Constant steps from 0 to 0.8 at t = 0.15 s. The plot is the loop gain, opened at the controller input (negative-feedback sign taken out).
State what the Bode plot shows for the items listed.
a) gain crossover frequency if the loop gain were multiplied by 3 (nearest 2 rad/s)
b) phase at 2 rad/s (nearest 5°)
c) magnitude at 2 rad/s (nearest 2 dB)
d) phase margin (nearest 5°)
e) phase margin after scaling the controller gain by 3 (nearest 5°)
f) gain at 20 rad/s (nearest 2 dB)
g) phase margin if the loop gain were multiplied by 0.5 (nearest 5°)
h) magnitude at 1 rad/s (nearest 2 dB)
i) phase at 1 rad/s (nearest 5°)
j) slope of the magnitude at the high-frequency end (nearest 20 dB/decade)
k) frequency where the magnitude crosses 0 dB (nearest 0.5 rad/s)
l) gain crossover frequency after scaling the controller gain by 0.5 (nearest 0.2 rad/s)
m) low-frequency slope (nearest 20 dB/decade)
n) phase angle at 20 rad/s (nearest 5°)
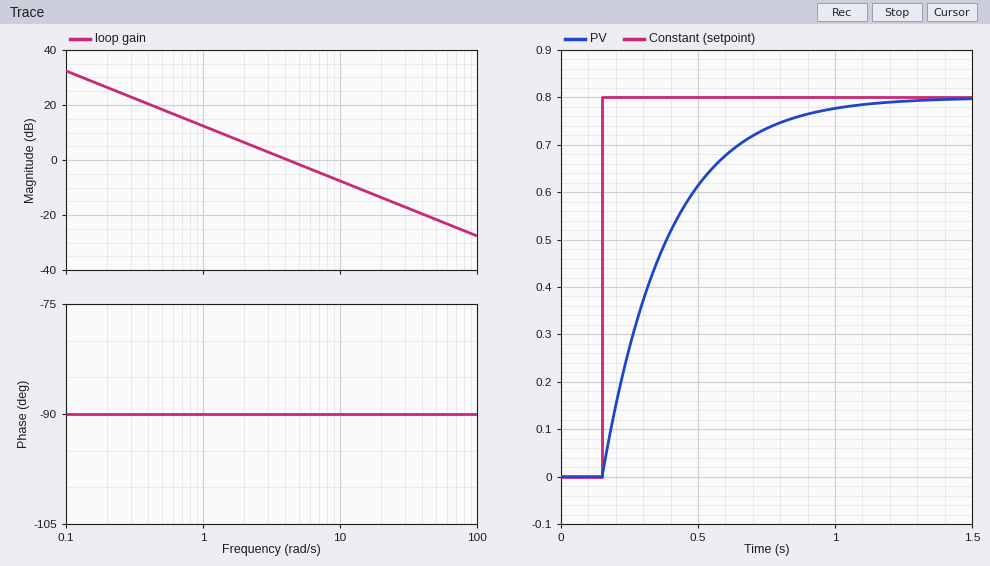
12 rad/s
-90°
6 dB
90°
90°
-14 dB
90°
12 dB
-90°
-20 dB/decade
4.0 rad/s
2.0 rad/s
-20 dB/decade
-90°
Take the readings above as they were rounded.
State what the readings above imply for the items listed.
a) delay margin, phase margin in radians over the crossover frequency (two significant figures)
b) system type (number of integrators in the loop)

0.39 s
1
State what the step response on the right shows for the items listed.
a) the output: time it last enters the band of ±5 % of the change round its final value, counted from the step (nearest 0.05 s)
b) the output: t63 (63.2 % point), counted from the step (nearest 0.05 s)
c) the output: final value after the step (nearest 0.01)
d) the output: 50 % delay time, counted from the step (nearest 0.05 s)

0.70 s
0.25 s
0.80
0.15 s
